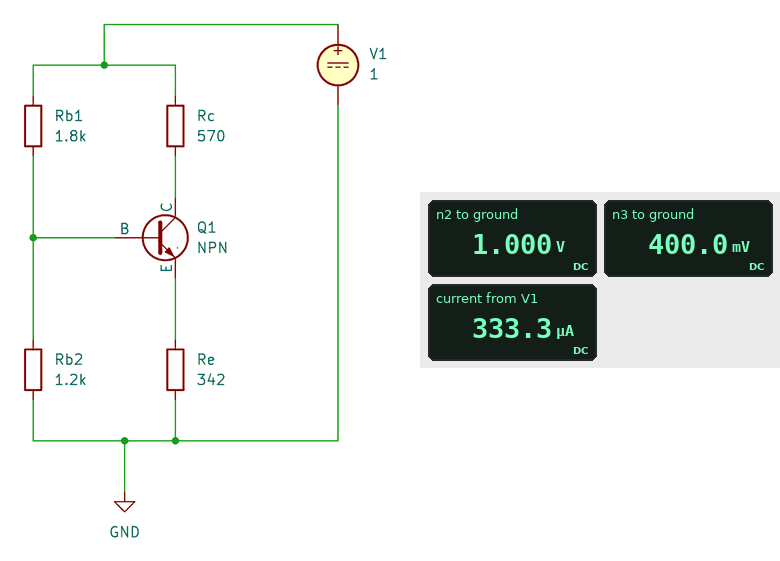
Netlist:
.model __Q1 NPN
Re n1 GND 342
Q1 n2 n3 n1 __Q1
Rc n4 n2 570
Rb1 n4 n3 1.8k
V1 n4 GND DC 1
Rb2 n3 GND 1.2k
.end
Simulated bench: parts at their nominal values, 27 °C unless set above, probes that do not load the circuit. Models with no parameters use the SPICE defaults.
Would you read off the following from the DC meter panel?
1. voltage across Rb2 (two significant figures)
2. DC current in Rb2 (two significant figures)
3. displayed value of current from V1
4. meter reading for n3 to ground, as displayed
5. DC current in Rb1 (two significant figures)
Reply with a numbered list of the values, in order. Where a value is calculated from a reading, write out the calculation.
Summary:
1. 400 mV = 400 mV
2. (400 mV) / 1.2 kΩ = 330 µA
3. 333.3 µA
4. 400.0 mV
5. (1 V - 400 mV) / 1.8 kΩ = 330 µA
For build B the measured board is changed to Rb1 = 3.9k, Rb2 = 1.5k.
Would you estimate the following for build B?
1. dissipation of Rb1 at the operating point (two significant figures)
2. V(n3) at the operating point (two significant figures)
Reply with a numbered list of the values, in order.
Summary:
1. 130 µW
2. 280 mV
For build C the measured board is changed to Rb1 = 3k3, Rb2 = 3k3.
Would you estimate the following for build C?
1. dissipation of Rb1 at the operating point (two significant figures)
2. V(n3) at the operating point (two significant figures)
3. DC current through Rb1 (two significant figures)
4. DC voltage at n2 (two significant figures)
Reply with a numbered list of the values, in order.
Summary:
1. 76 µW
2. 500 mV
3. 150 µA
4. 1.0 V
